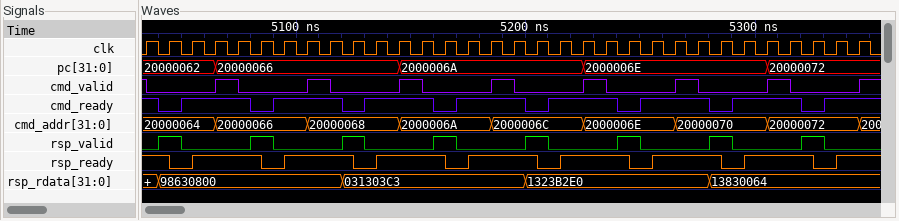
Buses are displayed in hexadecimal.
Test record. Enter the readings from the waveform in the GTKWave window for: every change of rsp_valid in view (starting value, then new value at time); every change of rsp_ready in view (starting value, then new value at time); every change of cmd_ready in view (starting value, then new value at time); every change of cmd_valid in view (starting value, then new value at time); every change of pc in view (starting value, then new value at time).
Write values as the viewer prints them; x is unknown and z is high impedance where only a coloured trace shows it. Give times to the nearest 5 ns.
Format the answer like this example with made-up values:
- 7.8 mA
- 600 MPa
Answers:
- 0, 1 at 5040 ns, 0 at 5050 ns, 1 at 5080 ns, 0 at 5090 ns, 1 at 5120 ns, 0 at 5130 ns, 1 at 5160 ns, 0 at 5170 ns, 1 at 5200 ns, 0 at 5210 ns, 1 at 5240 ns, 0 at 5250 ns, 1 at 5280 ns, 0 at 5290 ns, 1 at 5320 ns, 0 at 5330 ns
- 1, 0 at 5045 ns, 1 at 5055 ns, 0 at 5085 ns, 1 at 5095 ns, 0 at 5125 ns, 1 at 5135 ns, 0 at 5165 ns, 1 at 5175 ns, 0 at 5205 ns, 1 at 5215 ns, 0 at 5245 ns, 1 at 5255 ns, 0 at 5285 ns, 1 at 5295 ns, 0 at 5325 ns, 1 at 5335 ns
- 1, 0 at 5040 ns, 1 at 5050 ns, 0 at 5080 ns, 1 at 5090 ns, 0 at 5120 ns, 1 at 5130 ns, 0 at 5160 ns, 1 at 5170 ns, 0 at 5200 ns, 1 at 5210 ns, 0 at 5240 ns, 1 at 5250 ns, 0 at 5280 ns, 1 at 5290 ns, 0 at 5320 ns, 1 at 5330 ns
- 1, 0 at 5035 ns, 1 at 5065 ns, 0 at 5075 ns, 1 at 5105 ns, 0 at 5115 ns, 1 at 5145 ns, 0 at 5155 ns, 1 at 5185 ns, 0 at 5195 ns, 1 at 5225 ns, 0 at 5235 ns, 1 at 5265 ns, 0 at 5275 ns, 1 at 5305 ns, 0 at 5315 ns, 1 at 5345 ns
- 20000062, 20000066 at 5065 ns, 2000006A at 5145 ns, 2000006E at 5225 ns, 20000072 at 5305 ns
